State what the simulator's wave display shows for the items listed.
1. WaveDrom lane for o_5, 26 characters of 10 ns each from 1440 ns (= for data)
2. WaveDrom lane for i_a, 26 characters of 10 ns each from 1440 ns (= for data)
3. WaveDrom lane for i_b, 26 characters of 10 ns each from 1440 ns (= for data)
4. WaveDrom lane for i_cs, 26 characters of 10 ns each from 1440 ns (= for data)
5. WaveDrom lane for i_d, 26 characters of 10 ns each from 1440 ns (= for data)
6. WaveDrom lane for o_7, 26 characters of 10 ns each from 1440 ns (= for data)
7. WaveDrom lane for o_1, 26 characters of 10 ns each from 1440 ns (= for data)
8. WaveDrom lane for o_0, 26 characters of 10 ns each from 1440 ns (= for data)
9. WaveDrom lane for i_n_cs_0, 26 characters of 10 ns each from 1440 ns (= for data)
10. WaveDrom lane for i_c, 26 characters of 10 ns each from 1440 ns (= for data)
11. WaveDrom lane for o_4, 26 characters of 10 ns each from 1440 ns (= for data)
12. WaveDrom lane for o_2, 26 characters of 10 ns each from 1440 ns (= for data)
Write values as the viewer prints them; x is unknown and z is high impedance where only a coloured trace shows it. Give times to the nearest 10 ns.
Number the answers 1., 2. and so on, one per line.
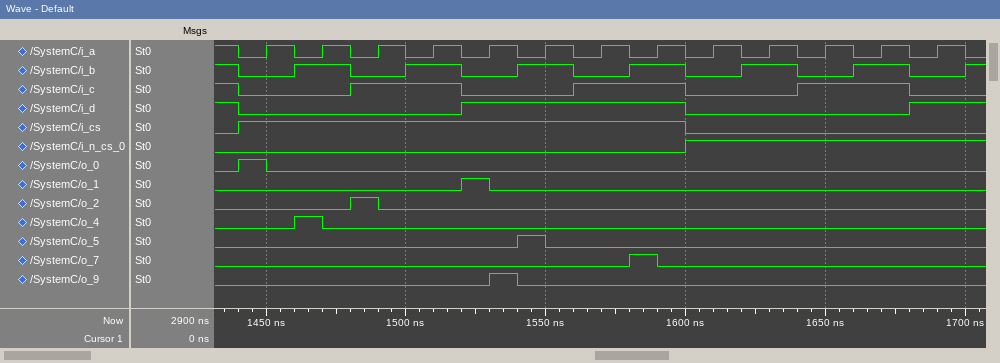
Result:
1. {name: 'o_5', wave: '0.........10..............'}
2. {name: 'i_a', wave: '01010101010101010101010101'}
3. {name: 'i_b', wave: '0.1.0.1.0.1.0.1.0.1.0.1.0.'}
4. {name: 'i_cs', wave: '1...............0.........'}
5. {name: 'i_d', wave: '0.......1.......0.......1.'}
6. {name: 'o_7', wave: '0.............10..........'}
7. {name: 'o_1', wave: '0.......10................'}
8. {name: 'o_0', wave: '10........................'}
9. {name: 'i_n_cs_0', wave: '0...............1.........'}
10. {name: 'i_c', wave: '0...1...0...1...0...1...0.'}
11. {name: 'o_4', wave: '0.10......................'}
12. {name: 'o_2', wave: '0...10....................'}
